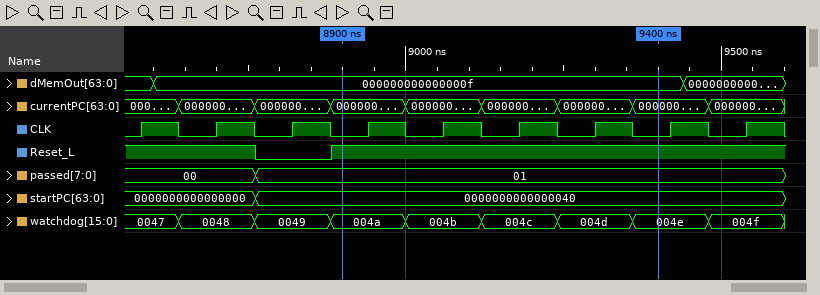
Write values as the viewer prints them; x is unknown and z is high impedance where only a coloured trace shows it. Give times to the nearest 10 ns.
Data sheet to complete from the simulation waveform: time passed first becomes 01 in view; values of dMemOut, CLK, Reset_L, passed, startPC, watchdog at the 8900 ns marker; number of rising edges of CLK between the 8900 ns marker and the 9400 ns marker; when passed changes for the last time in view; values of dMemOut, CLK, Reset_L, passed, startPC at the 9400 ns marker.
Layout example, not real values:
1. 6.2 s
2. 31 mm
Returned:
1. 8760 ns
2. dMemOut=000000000000000f, CLK=0, Reset_L=1, passed=01, startPC=0000000000000040, watchdog=004a
3. 4
4. 8760 ns
5. dMemOut=000000000000000f, CLK=0, Reset_L=1, passed=01, startPC=0000000000000040
